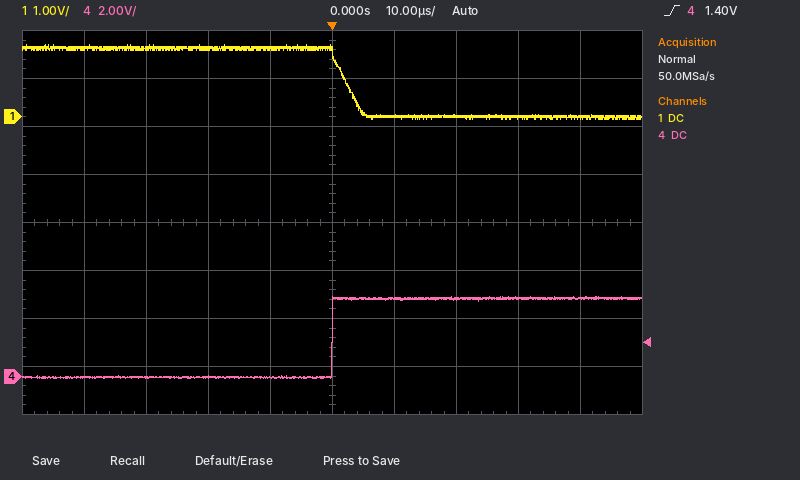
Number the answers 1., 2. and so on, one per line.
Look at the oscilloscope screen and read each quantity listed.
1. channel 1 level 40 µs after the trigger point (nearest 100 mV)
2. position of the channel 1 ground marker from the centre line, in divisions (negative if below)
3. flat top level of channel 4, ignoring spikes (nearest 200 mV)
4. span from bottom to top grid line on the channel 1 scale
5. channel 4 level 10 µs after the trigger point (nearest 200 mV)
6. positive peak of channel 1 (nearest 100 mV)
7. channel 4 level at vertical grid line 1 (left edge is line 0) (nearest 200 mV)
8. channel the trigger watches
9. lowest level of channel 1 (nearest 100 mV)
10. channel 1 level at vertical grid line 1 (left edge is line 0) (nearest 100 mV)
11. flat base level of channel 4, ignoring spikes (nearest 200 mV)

1. 0.0 V
2. +2.2 div
3. 3.2 V
4. 8 V
5. 3.2 V
6. 1.5 V
7. 0.0 V
8. channel 4
9. -100 mV
10. 1.4 V
11. 0.0 V
